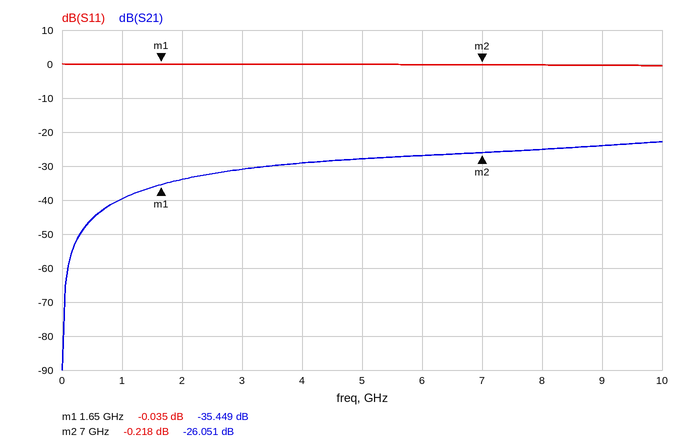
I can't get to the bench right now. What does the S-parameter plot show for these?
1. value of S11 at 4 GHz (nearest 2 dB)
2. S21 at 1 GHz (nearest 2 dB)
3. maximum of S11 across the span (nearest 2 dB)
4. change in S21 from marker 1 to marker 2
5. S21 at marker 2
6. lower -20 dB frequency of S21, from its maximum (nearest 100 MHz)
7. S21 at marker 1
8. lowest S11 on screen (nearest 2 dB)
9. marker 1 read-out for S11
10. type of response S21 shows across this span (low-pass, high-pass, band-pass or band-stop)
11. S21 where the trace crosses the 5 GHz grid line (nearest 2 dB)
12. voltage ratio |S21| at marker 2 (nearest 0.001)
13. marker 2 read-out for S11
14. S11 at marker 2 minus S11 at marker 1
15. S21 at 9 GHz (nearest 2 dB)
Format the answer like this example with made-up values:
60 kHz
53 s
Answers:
0 dB
-40 dB
0 dB
9.398 dB
-26.051 dB
700 MHz
-35.449 dB
0 dB
-0.035 dB
high-pass
-28 dB
0.050
-0.218 dB
-0.183 dB
-24 dB
